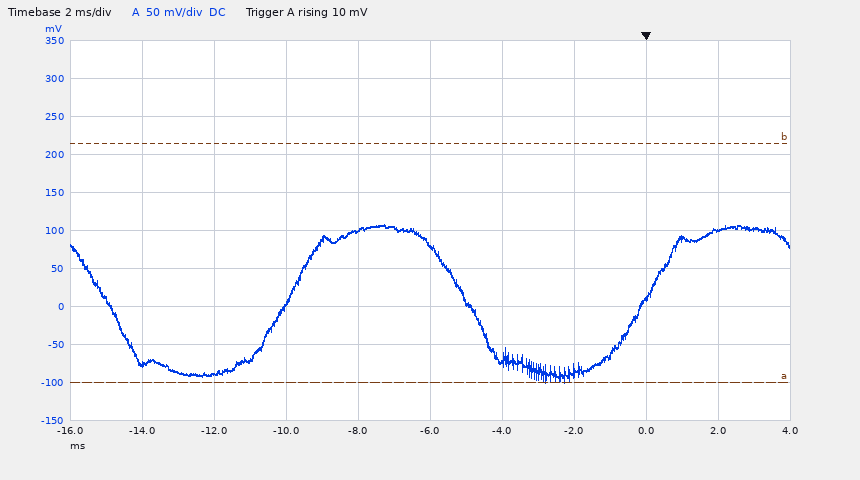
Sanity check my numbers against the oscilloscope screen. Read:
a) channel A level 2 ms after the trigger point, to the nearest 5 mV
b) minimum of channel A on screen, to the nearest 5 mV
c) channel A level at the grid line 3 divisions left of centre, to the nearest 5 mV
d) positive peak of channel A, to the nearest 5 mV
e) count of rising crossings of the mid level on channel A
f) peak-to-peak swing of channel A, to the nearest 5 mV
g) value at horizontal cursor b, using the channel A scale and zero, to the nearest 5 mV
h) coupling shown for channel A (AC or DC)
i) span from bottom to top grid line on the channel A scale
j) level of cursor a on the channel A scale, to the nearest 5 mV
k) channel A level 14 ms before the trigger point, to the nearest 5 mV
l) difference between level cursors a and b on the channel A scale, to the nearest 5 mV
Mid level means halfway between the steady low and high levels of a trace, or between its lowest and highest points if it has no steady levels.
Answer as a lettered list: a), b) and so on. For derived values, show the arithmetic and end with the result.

a) 100 mV
b) -100 mV
c) -90 mV
d) 110 mV
e) 2
f) 110 mV − (-100 mV) = 210 mV
g) 215 mV
h) DC
i) 500 mV
j) -100 mV
k) -75 mV
l) 315 mV
